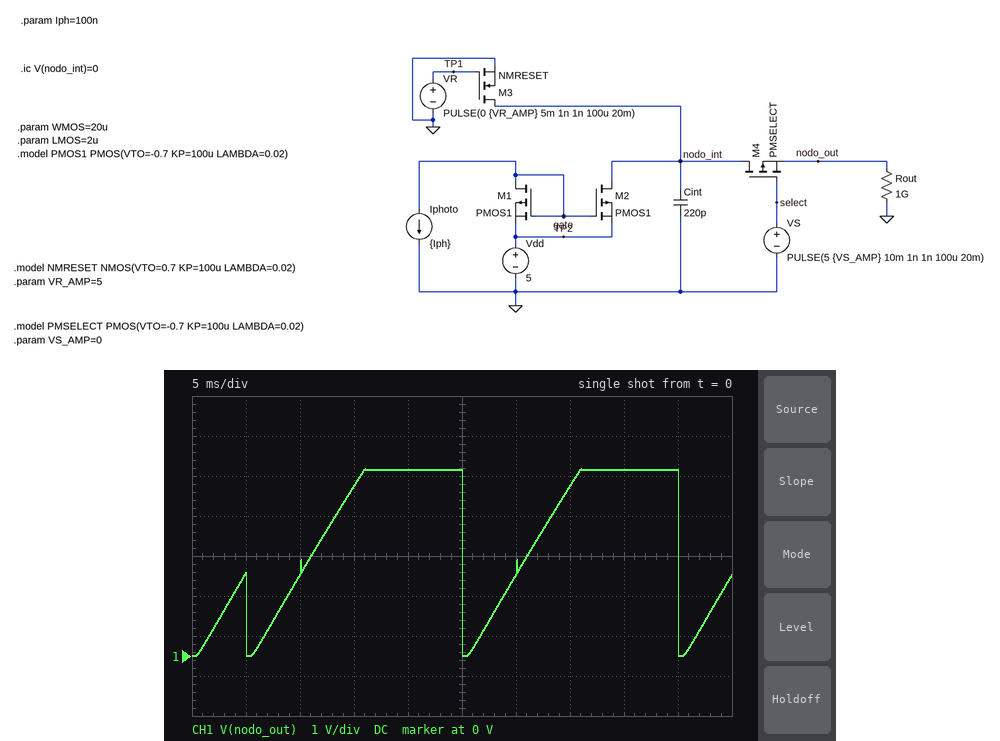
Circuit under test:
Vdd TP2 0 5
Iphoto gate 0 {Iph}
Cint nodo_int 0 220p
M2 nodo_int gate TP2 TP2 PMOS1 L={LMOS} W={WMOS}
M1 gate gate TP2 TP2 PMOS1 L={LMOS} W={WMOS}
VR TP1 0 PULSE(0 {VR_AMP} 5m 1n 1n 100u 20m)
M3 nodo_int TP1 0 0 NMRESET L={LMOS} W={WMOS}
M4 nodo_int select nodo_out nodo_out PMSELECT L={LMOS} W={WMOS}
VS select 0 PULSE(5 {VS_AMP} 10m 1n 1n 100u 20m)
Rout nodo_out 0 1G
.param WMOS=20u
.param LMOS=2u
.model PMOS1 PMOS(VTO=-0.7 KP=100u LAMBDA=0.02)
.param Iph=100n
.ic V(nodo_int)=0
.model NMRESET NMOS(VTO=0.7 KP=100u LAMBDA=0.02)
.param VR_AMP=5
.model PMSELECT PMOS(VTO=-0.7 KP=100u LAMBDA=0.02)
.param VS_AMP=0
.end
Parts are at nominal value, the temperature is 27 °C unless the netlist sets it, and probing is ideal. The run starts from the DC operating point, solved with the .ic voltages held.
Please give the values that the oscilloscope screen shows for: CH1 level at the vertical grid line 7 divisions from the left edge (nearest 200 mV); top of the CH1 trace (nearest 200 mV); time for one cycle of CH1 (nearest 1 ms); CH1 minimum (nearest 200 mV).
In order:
4.2 V
4.6 V
20 ms
0 V
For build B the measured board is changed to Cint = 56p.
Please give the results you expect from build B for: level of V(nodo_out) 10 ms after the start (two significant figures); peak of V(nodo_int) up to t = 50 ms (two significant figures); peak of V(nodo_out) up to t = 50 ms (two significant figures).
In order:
4.7 V
5.0 V
5.0 V
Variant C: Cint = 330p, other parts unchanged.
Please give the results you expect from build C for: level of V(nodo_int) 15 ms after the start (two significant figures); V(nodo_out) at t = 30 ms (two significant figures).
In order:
3.1 V
1.3 V
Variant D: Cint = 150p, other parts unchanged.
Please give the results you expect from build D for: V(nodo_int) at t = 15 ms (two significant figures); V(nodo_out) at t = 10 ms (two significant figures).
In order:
5.0 V
3.1 V
